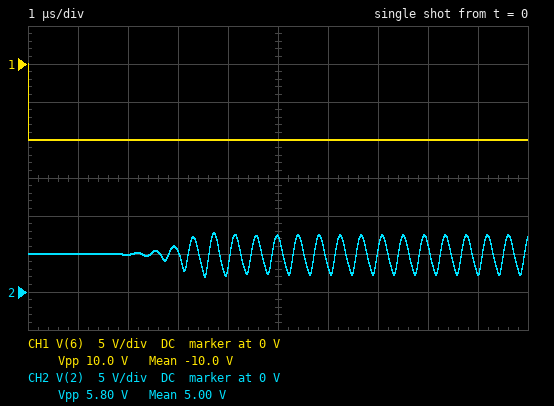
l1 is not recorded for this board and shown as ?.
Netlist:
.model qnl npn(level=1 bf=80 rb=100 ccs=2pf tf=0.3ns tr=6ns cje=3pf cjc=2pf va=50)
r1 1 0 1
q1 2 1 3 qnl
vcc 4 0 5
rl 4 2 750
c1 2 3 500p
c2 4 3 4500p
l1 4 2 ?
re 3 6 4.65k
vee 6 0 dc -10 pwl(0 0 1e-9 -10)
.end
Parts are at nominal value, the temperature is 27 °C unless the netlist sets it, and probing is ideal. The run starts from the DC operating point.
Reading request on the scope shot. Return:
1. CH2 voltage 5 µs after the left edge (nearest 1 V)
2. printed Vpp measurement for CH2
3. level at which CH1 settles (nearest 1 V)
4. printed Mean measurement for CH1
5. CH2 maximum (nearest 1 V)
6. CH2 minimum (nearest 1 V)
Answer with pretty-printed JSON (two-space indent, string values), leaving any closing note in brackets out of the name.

{
  "CH2 voltage 5 µs after the left edge": "7 V",
  "printed Vpp measurement for CH2": "5.80 V",
  "level at which CH1 settles": "-10 V",
  "printed Mean measurement for CH1": "-10.0 V",
  "CH2 maximum": "8 V",
  "CH2 minimum": "2 V"
}
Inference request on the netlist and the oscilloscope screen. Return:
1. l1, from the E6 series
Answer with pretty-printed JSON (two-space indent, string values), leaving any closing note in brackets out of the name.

{
  "l1, from the E6 series": "10 µH"
}
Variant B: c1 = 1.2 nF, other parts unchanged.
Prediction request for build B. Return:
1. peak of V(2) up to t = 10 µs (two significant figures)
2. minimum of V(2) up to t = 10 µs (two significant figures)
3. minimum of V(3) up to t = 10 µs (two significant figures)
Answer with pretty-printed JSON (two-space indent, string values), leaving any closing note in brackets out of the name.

{
  "peak of V(2) up to t = 10 µs": "7.8 V",
  "minimum of V(2) up to t = 10 µs": "2.1 V",
  "minimum of V(3) up to t = 10 µs": "-910 mV"
}
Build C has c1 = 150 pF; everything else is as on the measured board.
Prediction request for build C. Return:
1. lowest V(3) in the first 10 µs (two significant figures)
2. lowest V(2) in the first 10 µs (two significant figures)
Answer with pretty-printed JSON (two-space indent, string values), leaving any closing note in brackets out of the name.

{
  "lowest V(3) in the first 10 µs": "-830 mV",
  "lowest V(2) in the first 10 µs": "2.9 V"
}
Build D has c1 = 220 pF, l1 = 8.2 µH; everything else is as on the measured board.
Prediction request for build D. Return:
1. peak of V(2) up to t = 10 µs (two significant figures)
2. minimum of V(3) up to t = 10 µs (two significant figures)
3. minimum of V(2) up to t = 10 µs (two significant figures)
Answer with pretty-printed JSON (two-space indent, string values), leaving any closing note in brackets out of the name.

{
  "peak of V(2) up to t = 10 µs": "7.4 V",
  "minimum of V(3) up to t = 10 µs": "-850 mV",
  "minimum of V(2) up to t = 10 µs": "2.4 V"
}
